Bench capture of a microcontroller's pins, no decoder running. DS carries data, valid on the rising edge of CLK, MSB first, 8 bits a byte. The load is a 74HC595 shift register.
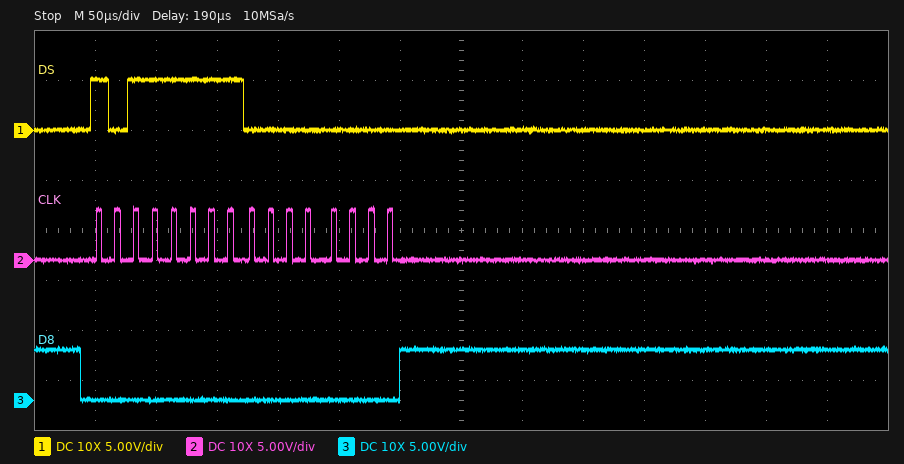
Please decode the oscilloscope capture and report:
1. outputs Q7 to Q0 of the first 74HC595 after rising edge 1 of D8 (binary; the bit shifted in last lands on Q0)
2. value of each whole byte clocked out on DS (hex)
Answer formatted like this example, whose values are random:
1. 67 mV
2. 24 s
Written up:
1. 00000000
2. BF 00
